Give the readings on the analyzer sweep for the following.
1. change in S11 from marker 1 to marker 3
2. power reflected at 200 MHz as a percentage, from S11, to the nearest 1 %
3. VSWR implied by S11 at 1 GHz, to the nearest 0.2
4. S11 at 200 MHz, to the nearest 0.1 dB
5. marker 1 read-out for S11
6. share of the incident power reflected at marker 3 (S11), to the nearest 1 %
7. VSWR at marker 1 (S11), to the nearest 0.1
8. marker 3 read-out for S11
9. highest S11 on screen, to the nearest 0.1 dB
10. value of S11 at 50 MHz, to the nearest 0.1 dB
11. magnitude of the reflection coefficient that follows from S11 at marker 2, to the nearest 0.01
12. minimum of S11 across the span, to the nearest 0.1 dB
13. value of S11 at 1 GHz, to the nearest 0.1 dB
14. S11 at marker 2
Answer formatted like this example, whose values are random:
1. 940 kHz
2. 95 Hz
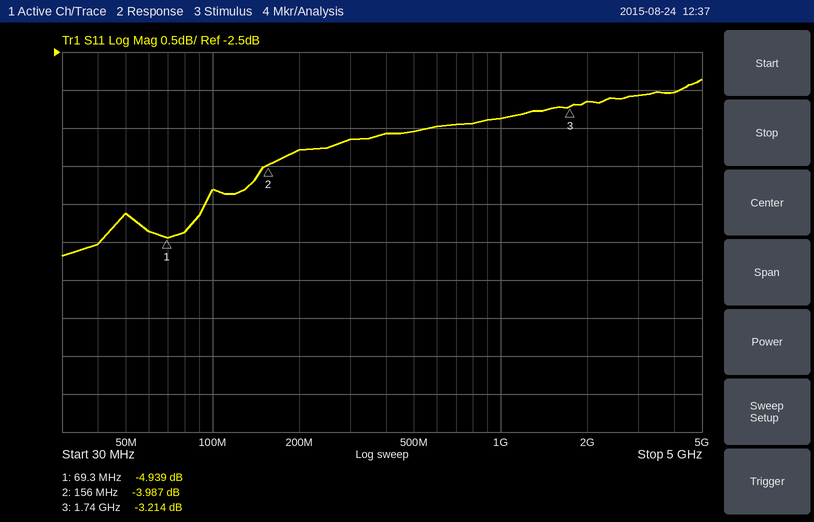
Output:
1. 1.725 dB
2. 42 %
3. 5.2
4. -3.8 dB
5. -4.939 dB
6. 48 %
7. 3.6
8. -3.214 dB
9. -2.9 dB
10. -4.6 dB
11. 0.63
12. -5.2 dB
13. -3.4 dB
14. -3.987 dB
